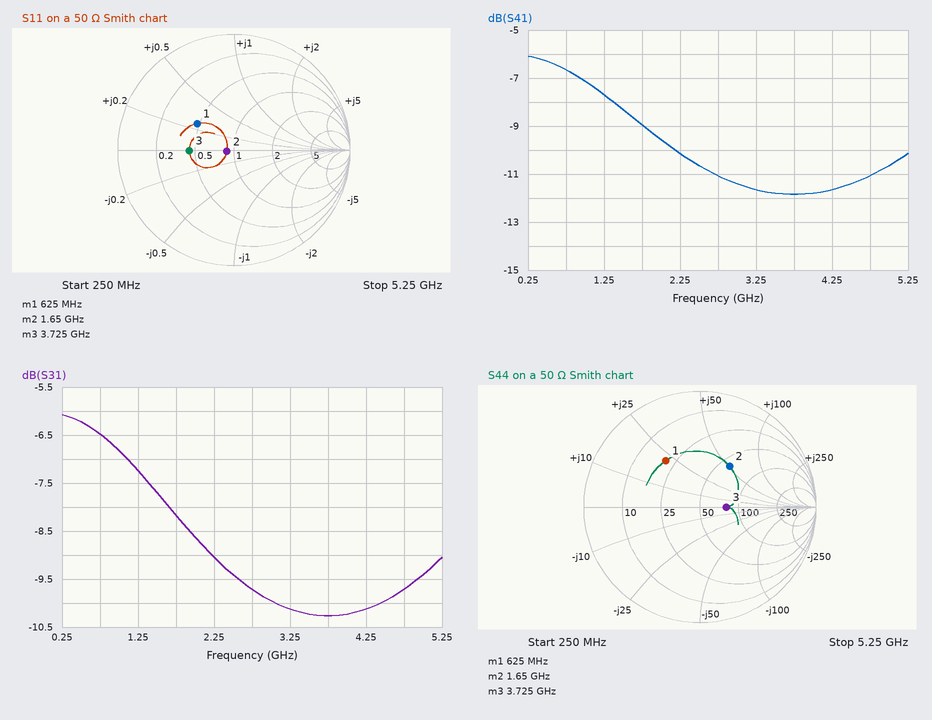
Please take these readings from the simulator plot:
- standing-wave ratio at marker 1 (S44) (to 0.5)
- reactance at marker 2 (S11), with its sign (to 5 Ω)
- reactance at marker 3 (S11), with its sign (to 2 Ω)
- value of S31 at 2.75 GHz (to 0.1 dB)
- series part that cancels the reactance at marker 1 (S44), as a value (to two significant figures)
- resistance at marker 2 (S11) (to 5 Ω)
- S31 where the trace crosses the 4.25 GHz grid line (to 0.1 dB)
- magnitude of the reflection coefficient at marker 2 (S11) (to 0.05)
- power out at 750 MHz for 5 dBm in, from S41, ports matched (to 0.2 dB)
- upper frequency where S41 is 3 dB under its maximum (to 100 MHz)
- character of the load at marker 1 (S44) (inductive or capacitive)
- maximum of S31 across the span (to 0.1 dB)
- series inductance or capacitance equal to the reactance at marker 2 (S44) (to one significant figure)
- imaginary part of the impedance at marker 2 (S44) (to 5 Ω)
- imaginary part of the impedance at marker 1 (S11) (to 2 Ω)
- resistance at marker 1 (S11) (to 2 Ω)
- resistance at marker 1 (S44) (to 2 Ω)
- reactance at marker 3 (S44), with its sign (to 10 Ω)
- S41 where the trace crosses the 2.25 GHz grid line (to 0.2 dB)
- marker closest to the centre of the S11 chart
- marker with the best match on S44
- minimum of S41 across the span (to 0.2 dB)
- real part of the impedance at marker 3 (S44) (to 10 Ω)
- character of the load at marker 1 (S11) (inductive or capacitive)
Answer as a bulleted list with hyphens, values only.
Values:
- 3.0
- 0 Ω
- 0 Ω
- -9.7 dB
- 12 pF
- 45 Ω
- -10.1 dB
- 0.05
- -1.6 dBm
- 1.8 GHz
- inductive
- -6.1 dB
- 5 nH
- +50 Ω
- +12 Ω
- 24 Ω
- 20 Ω
- 0 Ω
- -10.2 dB
- marker 2
- marker 3
- -11.8 dB
- 80 Ω
- inductive
